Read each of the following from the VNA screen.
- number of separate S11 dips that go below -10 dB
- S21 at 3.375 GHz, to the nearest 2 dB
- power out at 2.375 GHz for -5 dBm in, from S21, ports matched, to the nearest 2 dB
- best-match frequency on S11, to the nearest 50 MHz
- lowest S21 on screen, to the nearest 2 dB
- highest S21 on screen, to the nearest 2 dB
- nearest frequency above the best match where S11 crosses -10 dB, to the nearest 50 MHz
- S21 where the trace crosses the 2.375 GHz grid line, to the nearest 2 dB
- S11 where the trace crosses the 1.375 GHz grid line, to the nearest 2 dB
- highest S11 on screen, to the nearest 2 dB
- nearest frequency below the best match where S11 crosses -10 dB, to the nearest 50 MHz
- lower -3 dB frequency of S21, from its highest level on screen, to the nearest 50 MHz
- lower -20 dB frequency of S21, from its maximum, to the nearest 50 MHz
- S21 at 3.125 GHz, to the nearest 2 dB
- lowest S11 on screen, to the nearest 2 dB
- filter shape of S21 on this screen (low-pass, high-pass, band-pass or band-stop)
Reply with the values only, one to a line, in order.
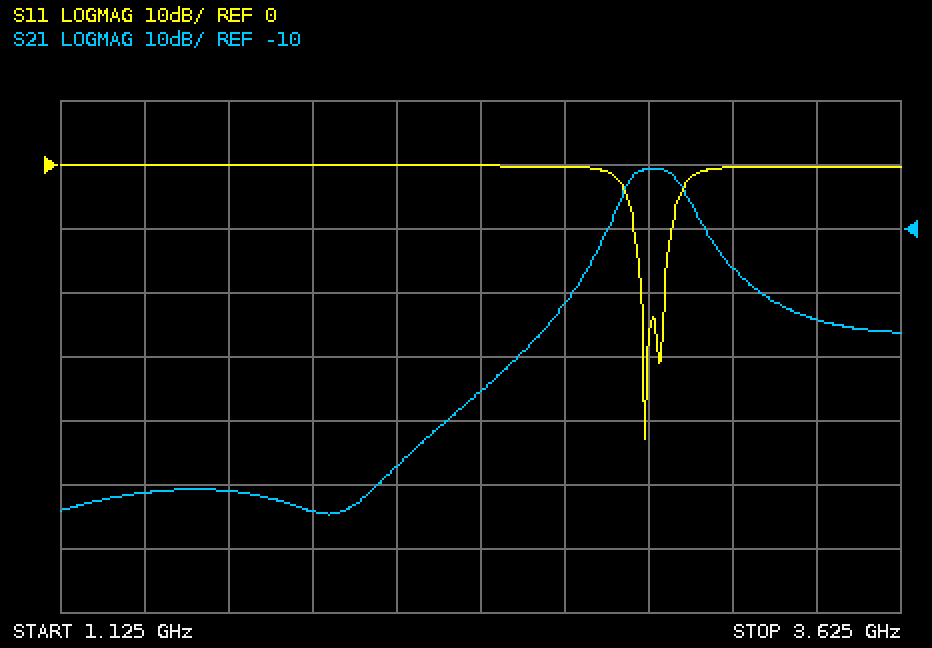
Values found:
2
-24 dB
-40 dBm
2.85 GHz
-54 dB
0 dB
2.95 GHz
-36 dB
0 dB
0 dB
2.85 GHz
2.80 GHz
2.65 GHz
-16 dB
-42 dB
band-pass
